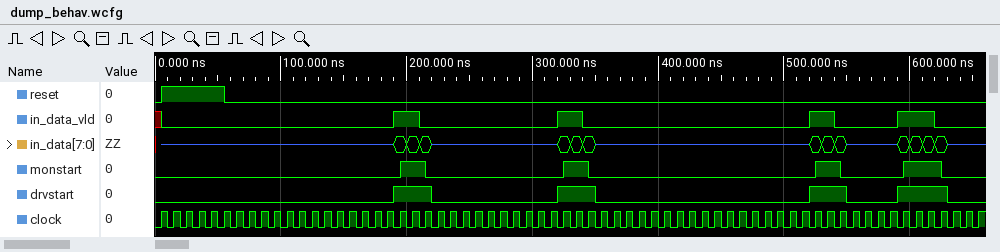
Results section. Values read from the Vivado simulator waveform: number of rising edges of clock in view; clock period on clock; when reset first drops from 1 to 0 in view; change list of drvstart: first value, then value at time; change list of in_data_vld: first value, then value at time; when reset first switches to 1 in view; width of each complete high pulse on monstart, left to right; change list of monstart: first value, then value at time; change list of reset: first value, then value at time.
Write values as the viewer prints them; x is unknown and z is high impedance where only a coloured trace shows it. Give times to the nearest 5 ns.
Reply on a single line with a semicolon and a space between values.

66; 10 ns; 55 ns; 0, 1 at 190 ns, 0 at 220 ns, 1 at 320 ns, 0 at 350 ns, 1 at 520 ns, 0 at 550 ns, 1 at 590 ns, 0 at 630 ns; x, 0 at 5 ns, 1 at 190 ns, 0 at 210 ns, 1 at 320 ns, 0 at 340 ns, 1 at 520 ns, 0 at 540 ns, 1 at 590 ns, 0 at 620 ns; 5 ns; 20 ns, 20 ns, 20 ns, 30 ns; 0, 1 at 195 ns, 0 at 215 ns, 1 at 325 ns, 0 at 345 ns, 1 at 525 ns, 0 at 545 ns, 1 at 595 ns, 0 at 625 ns; 0, 1 at 5 ns, 0 at 55 ns
